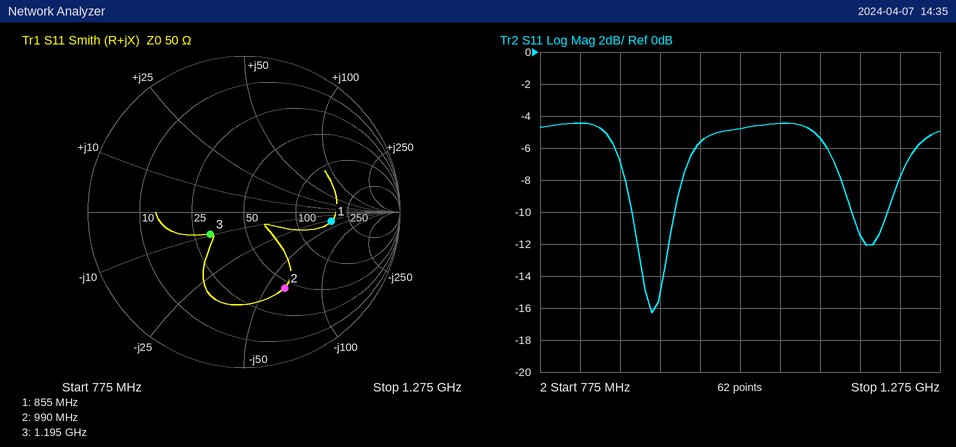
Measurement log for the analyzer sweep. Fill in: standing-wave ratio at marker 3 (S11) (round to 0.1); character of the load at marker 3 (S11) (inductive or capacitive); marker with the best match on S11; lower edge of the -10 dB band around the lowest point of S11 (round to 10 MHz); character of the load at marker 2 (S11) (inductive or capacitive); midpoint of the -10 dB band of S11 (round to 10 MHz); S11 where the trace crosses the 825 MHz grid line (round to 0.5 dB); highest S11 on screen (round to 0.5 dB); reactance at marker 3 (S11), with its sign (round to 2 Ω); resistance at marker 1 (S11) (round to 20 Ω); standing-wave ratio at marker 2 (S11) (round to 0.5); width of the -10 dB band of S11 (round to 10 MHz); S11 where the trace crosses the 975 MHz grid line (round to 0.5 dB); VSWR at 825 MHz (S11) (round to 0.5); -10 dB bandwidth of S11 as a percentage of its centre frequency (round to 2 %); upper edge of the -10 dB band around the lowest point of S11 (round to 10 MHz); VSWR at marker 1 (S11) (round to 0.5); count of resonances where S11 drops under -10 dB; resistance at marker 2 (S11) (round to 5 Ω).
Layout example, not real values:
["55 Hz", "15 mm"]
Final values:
["1.7", "capacitive", "marker 3", "890 MHz", "capacitive", "920 MHz", "-4.5 dB", "-4.5 dB", "-10 Ω", "180 Ω", "3.5", "50 MHz", "-5.5 dB", "4.0", "6 %", "940 MHz", "3.5", "2", "45 Ω"]
